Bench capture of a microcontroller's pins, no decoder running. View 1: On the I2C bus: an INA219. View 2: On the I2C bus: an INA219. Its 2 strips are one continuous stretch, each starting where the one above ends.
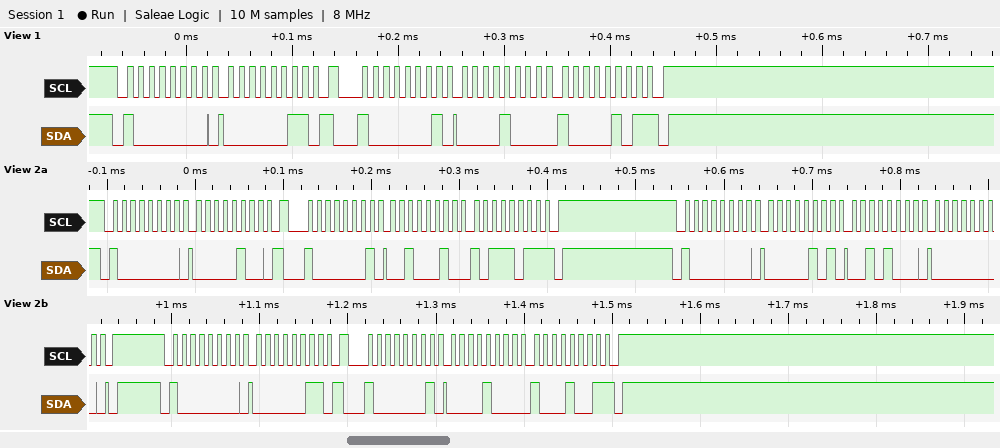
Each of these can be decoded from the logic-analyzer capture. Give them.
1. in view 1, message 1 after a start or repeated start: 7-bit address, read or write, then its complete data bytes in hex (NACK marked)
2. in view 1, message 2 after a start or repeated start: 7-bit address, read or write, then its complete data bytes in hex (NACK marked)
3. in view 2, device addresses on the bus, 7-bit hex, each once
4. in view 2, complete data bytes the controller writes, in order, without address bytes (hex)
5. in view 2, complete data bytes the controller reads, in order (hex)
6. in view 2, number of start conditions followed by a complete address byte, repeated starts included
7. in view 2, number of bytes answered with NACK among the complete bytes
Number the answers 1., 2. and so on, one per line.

1. 0x40 write: 03
2. 0x40 read: 08 85 NACK
3. 0x40
4. 04 05 28 00 03
5. 22 BB 08 89
6. 5
7. 2
